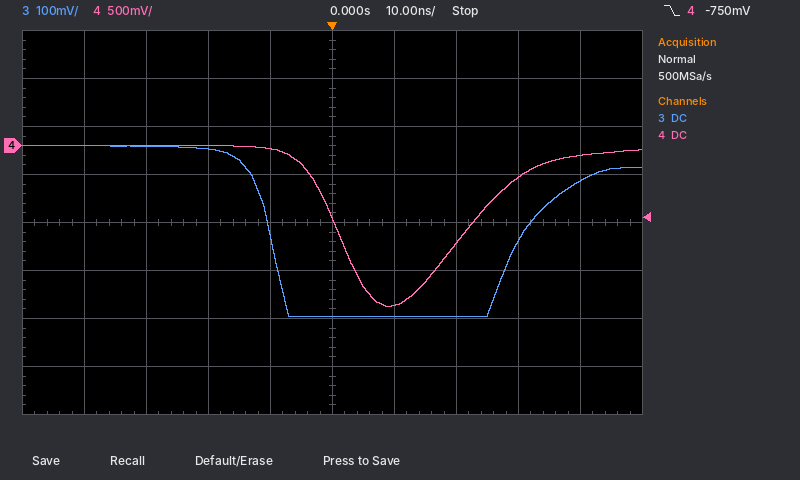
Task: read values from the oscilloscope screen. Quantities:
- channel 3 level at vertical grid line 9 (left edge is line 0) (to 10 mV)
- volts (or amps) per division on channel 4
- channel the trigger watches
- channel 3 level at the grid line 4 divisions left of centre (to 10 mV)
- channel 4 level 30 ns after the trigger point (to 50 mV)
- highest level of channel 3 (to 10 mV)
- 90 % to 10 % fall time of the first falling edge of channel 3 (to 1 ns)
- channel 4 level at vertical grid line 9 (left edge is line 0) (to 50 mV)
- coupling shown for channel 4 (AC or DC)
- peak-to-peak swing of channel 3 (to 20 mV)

-70 mV
500 mV
channel 4
0 mV
-350 mV
0 mV
7 ns
-100 mV
DC
360 mV
